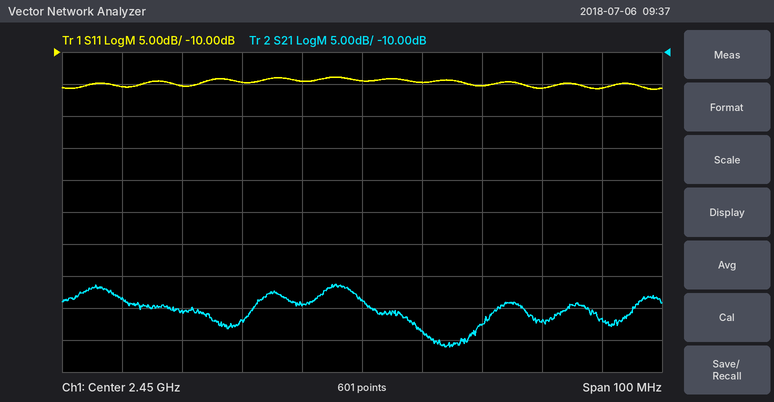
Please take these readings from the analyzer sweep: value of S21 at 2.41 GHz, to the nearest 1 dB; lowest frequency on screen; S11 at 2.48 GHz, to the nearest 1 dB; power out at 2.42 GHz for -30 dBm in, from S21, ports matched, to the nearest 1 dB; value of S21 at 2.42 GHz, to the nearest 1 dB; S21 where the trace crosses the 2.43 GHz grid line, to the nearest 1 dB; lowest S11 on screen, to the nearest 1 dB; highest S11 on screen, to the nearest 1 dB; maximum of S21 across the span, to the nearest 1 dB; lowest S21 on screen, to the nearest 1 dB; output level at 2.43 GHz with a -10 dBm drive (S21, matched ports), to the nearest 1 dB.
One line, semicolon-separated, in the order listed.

-48 dB; 2.4 GHz; -16 dB; -80 dBm; -50 dB; -52 dB; -16 dB; -14 dB; -46 dB; -56 dB; -62 dBm
